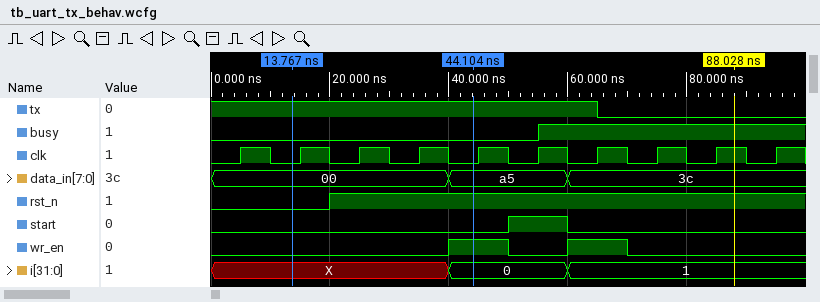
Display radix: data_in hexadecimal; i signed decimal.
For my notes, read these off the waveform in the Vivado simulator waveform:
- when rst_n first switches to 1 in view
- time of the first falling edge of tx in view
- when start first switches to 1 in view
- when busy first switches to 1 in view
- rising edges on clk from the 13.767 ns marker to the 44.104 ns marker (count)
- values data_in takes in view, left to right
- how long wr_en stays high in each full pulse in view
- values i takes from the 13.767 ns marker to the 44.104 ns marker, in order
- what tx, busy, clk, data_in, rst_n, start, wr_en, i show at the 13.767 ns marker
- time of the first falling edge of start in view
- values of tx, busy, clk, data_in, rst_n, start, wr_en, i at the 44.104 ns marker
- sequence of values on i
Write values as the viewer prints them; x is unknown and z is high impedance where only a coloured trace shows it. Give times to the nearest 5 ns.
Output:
20 ns
65 ns
50 ns
55 ns
3
00, a5, 3c
10 ns, 10 ns
X, 0
tx=1, busy=0, clk=0, data_in=00, rst_n=0, start=0, wr_en=0, i=X
60 ns
tx=1, busy=0, clk=0, data_in=a5, rst_n=1, start=0, wr_en=1, i=0
X, 0, 1
